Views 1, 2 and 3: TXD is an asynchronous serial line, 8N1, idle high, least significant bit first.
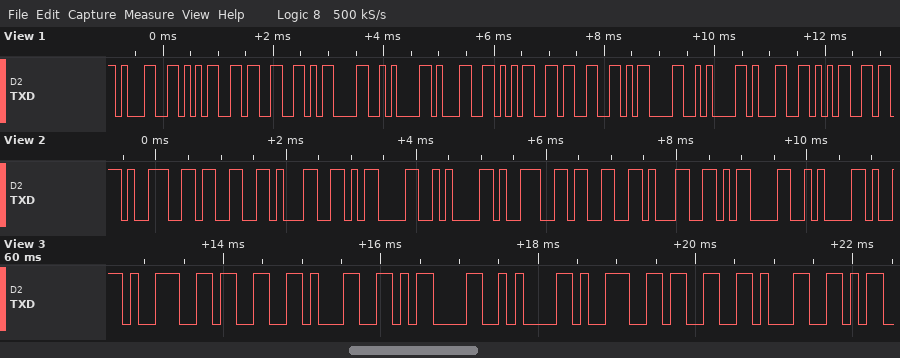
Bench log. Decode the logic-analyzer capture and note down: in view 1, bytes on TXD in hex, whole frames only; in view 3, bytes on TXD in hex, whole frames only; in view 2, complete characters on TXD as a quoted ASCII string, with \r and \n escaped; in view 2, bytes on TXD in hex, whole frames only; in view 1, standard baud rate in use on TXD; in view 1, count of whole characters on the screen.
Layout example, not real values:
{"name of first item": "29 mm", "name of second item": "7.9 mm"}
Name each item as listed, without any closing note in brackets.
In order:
{"in view 1, bytes on TXD in hex, whole frames only": "31 35 33 0D 0A 31 35 33 0D 0A 31 35", "in view 3, bytes on TXD in hex, whole frames only": "39 33 31 0D 0A 39 33 31", "in view 2, complete characters on TXD as a quoted ASCII string, with \\r and \\n escaped": "\"931\\r\\n931\\r\\n\"", "in view 2, bytes on TXD in hex, whole frames only": "39 33 31 0D 0A 39 33 31 0D 0A", "in view 1, standard baud rate in use on TXD": "9600 baud", "in view 1, count of whole characters on the screen": "12"}
